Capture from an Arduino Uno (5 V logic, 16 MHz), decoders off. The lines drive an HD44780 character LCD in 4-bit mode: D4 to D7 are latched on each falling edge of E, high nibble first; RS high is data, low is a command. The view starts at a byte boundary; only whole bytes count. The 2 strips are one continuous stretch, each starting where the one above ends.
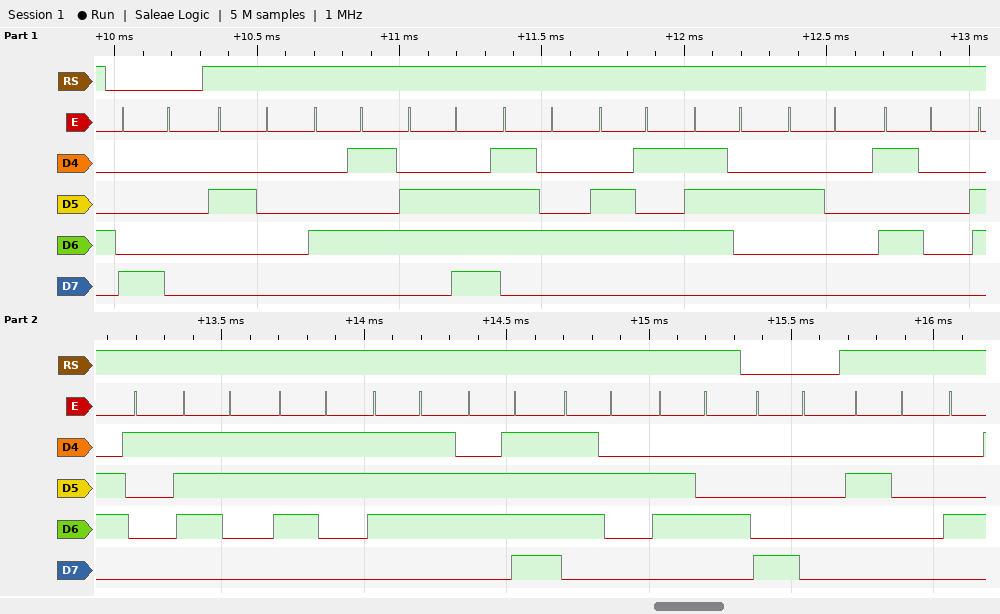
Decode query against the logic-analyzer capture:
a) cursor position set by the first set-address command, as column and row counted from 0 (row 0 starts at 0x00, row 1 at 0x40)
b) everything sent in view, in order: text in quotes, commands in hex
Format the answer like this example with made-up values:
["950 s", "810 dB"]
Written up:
["column 0, row 0", "0x80 \" Enter Password\" 0x80 \" \""]
